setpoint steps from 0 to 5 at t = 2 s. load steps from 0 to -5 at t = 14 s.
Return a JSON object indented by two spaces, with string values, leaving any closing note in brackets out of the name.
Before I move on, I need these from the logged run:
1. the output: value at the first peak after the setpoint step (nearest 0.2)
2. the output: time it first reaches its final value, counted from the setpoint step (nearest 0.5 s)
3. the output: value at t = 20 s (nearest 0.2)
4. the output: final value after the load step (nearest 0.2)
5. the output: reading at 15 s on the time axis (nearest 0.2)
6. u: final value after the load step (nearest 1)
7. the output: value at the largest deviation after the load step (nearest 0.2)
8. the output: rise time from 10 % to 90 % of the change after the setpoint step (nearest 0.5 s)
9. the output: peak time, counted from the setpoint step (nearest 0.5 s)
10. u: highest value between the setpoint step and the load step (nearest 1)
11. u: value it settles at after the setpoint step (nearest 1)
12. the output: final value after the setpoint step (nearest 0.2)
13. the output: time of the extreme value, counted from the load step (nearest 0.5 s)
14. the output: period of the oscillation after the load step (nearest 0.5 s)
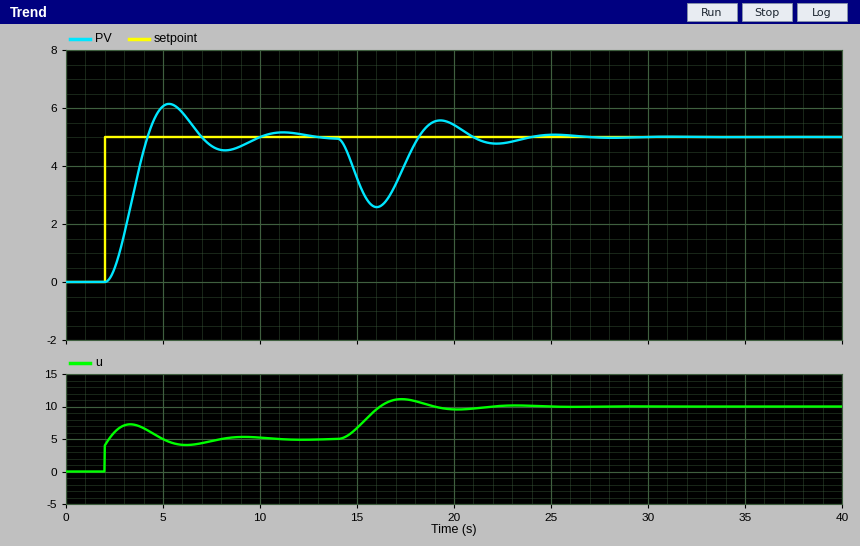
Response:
{
  "the output: value at the first peak after the setpoint step": "6.2",
  "the output: time it first reaches its final value, counted from the setpoint step": "2.0 s",
  "the output: value at t = 20 s": "5.4",
  "the output: final value after the load step": "5.0",
  "the output: reading at 15 s on the time axis": "3.6",
  "u: final value after the load step": "10",
  "the output: value at the largest deviation after the load step": "2.6",
  "the output: rise time from 10 % to 90 % of the change after the setpoint step": "1.5 s",
  "the output: peak time, counted from the setpoint step": "3.5 s",
  "u: highest value between the setpoint step and the load step": "7",
  "u: value it settles at after the setpoint step": "5",
  "the output: final value after the setpoint step": "5.0",
  "the output: time of the extreme value, counted from the load step": "2.0 s",
  "the output: period of the oscillation after the load step": "6.0 s"
}
